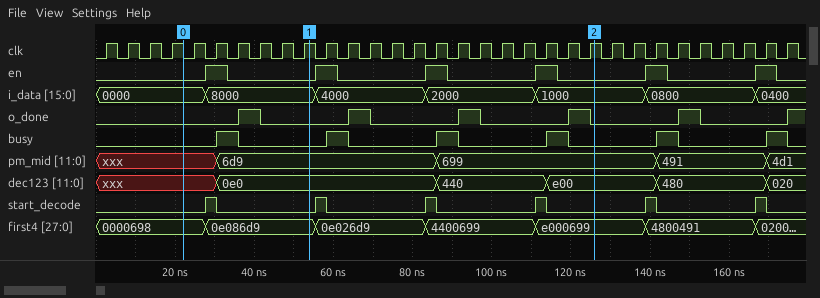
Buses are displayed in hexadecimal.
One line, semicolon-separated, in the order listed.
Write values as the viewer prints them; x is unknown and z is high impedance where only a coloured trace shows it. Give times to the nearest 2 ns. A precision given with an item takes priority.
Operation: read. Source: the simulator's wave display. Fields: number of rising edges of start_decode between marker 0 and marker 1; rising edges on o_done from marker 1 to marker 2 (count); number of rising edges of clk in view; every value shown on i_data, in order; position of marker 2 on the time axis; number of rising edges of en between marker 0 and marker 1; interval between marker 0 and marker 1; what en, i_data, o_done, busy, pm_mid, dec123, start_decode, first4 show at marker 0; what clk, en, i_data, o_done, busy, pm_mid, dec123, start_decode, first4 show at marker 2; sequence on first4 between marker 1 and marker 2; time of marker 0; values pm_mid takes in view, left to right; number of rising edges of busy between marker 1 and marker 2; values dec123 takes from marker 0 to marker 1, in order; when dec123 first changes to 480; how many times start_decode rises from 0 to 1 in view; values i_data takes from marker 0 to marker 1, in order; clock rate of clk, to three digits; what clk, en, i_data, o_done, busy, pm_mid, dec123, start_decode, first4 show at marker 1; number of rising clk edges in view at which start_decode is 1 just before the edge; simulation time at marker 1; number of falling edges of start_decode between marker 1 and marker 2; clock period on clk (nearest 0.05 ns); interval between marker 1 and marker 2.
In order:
1; 3; 32; 0000, 8000, 4000, 2000, 1000, 0800, 0400; 126 ns; 1; 32 ns; en=0, i_data=0000, o_done=0, busy=0, pm_mid=xxx, dec123=xxx, start_decode=0, first4=0000698; clk=1, en=0, i_data=1000, o_done=0, busy=0, pm_mid=699, dec123=e00, start_decode=0, first4=e000699; 0e086d9, 0e026d9, 4400699, e000699; 22 ns; xxx, 6d9, 699, 491, 4d1; 3; xxx, 0e0; 142 ns; 6; 0000, 8000; 180 MHz; clk=1, en=0, i_data=8000, o_done=0, busy=0, pm_mid=6d9, dec123=0e0, start_decode=0, first4=0e086d9; 6; 54 ns; 3; 5.55 ns; 72 ns
